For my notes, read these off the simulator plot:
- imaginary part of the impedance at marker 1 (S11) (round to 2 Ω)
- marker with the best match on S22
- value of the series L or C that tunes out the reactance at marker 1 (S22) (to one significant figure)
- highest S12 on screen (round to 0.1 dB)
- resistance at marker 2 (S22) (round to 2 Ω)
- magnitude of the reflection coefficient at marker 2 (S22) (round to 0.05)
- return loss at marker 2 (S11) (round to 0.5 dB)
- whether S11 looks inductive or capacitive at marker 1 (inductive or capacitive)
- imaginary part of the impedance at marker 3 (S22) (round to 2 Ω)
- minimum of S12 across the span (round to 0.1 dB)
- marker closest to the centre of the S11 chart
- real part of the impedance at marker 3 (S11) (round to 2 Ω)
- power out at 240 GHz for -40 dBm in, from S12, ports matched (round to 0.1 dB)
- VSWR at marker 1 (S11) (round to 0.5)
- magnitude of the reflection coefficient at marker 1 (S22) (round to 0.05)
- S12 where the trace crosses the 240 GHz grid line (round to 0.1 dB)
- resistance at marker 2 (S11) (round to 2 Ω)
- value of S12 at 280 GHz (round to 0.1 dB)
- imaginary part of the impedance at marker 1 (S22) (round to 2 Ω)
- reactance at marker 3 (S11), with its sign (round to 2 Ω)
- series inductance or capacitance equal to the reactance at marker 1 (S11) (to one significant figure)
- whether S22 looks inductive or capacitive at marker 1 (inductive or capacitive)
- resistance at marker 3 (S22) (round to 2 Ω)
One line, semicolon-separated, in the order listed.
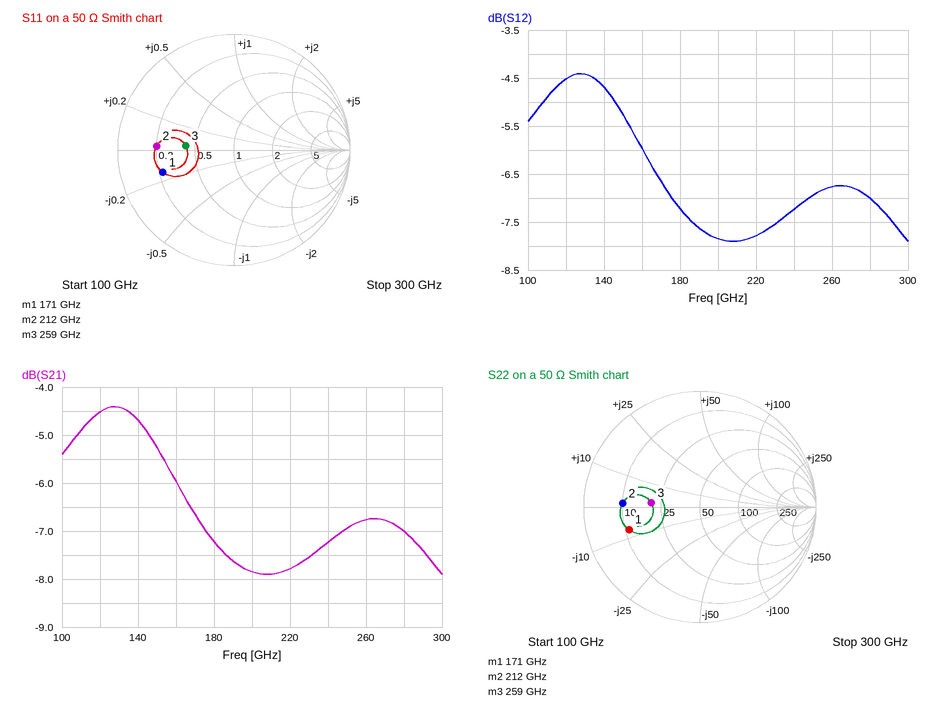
-8 Ω; marker 3; 7 pH; -4.4 dB; 10 Ω; 0.65; 3.5 dB; capacitive; +2 Ω; -7.9 dB; marker 3; 20 Ω; -47.2 dBm; 4.5; 0.65; -7.2 dB; 10 Ω; -7.0 dB; -8 Ω; +2 Ω; 100 fF; capacitive; 20 Ω
